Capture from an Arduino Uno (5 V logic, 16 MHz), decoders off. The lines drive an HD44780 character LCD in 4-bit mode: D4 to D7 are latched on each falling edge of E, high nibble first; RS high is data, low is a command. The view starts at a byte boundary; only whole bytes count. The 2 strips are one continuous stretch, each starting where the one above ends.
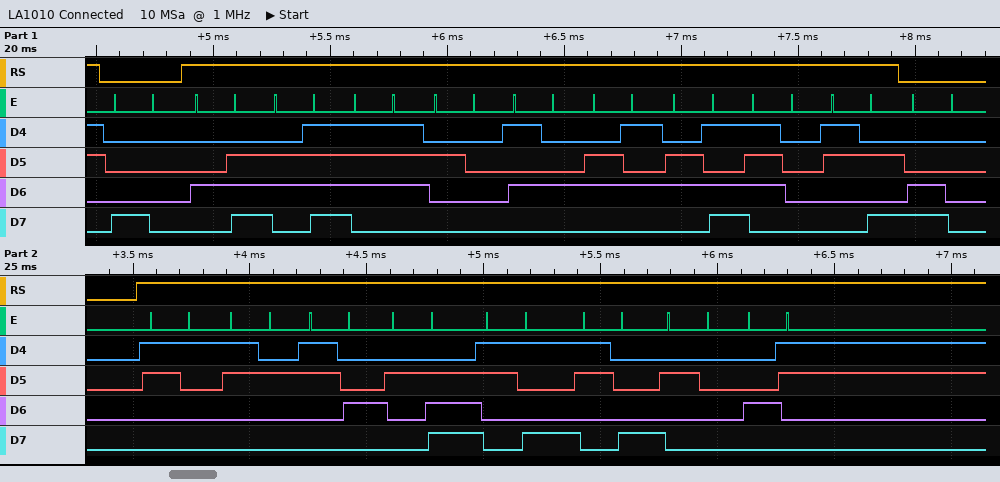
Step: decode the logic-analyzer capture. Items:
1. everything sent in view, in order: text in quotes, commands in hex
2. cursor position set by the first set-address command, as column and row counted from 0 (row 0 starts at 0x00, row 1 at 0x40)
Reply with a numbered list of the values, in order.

1. 0x80 "Now Temp:" 0xC0 "124.98 C"
2. column 0, row 0
